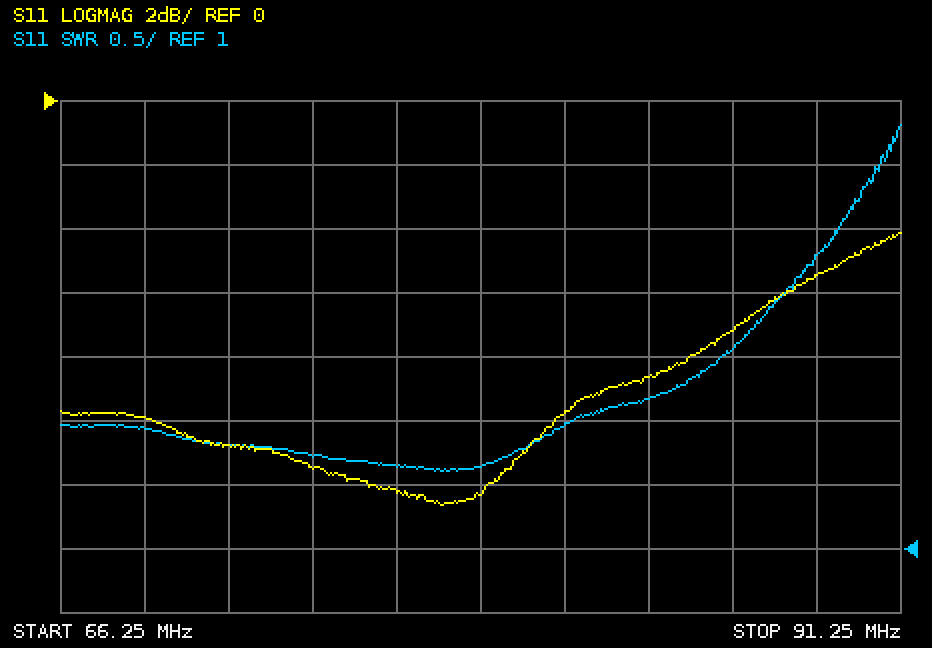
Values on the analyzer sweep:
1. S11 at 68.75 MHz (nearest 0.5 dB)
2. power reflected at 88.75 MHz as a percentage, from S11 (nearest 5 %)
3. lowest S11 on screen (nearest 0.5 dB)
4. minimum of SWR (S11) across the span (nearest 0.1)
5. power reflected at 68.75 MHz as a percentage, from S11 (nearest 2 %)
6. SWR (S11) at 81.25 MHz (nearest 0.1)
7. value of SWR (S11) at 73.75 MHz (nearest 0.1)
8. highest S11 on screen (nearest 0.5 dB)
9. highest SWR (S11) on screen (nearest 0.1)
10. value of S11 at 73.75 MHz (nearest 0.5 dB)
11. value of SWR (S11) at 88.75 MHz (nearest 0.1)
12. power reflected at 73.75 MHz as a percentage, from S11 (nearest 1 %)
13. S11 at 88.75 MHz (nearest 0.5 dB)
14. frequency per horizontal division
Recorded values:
-10.0 dB
30 %
-12.5 dB
1.6
10 %
2.0
1.7
-4.0 dB
4.3
-11.5 dB
3.3
7 %
-5.5 dB
2.5 MHz
